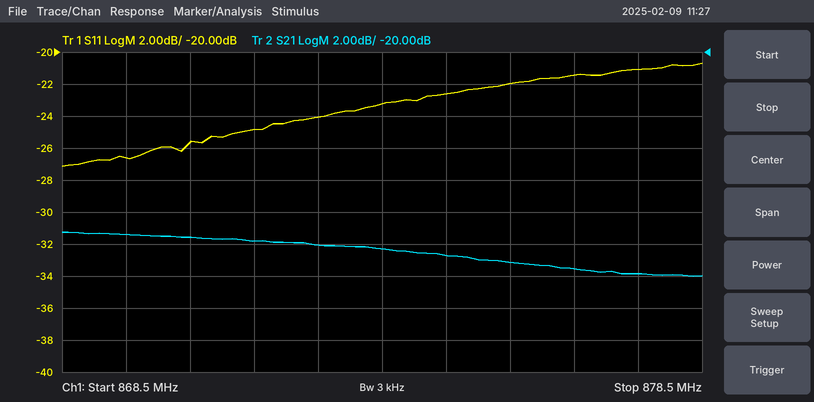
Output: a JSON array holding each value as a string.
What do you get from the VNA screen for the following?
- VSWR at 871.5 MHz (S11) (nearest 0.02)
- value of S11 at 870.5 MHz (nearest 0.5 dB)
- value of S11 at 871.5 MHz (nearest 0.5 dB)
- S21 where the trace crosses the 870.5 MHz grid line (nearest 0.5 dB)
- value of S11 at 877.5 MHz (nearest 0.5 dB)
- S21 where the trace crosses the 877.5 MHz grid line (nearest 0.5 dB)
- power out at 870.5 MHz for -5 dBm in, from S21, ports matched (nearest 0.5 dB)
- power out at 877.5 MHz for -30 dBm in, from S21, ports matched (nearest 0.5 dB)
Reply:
["1.12", "-25.5 dB", "-25.0 dB", "-31.5 dB", "-21.0 dB", "-34.0 dB", "-36.5 dBm", "-64.0 dBm"]
